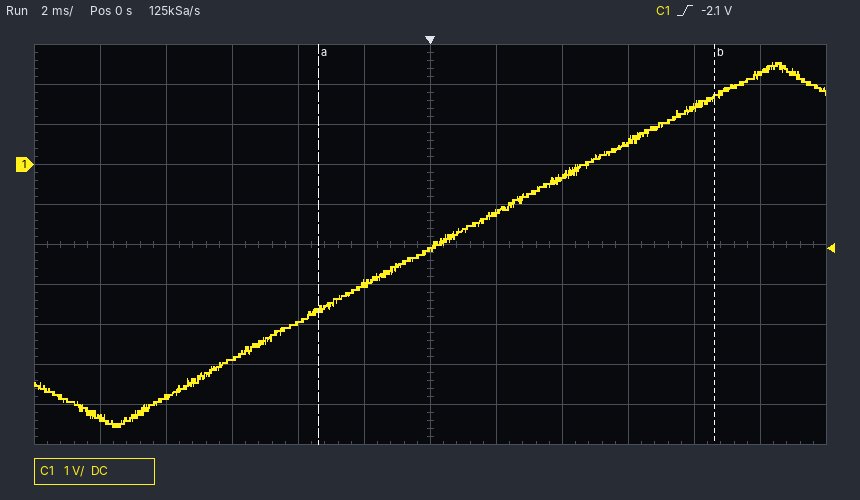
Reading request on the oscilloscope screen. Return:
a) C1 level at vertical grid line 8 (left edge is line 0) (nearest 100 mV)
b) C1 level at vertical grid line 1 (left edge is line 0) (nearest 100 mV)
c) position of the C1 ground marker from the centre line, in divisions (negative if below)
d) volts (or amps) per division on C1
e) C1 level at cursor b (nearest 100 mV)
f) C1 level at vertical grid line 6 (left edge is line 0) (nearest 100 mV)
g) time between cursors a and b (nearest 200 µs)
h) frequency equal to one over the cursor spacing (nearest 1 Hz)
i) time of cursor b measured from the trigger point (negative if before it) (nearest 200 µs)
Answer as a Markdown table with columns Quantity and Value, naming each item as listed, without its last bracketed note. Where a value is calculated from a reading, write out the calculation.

| Quantity | Value |
|---|---|
| C1 level at vertical grid line 8 (left edge is line 0) | -300 mV |
| C1 level at vertical grid line 1 (left edge is line 0) | -6.3 V |
| position of the C1 ground marker from the centre line, in divisions | +2.0 div |
| volts (or amps) per division on C1 | 1 V |
| C1 level at cursor b | 1.7 V |
| C1 level at vertical grid line 6 (left edge is line 0) | -2.1 V |
| time between cursors a and b | 12.0 ms |
| frequency equal to one over the cursor spacing | 1 / 12.0 ms ≈ 83 Hz |
| time of cursor b measured from the trigger point (negative if before it) | +8.6 ms |
